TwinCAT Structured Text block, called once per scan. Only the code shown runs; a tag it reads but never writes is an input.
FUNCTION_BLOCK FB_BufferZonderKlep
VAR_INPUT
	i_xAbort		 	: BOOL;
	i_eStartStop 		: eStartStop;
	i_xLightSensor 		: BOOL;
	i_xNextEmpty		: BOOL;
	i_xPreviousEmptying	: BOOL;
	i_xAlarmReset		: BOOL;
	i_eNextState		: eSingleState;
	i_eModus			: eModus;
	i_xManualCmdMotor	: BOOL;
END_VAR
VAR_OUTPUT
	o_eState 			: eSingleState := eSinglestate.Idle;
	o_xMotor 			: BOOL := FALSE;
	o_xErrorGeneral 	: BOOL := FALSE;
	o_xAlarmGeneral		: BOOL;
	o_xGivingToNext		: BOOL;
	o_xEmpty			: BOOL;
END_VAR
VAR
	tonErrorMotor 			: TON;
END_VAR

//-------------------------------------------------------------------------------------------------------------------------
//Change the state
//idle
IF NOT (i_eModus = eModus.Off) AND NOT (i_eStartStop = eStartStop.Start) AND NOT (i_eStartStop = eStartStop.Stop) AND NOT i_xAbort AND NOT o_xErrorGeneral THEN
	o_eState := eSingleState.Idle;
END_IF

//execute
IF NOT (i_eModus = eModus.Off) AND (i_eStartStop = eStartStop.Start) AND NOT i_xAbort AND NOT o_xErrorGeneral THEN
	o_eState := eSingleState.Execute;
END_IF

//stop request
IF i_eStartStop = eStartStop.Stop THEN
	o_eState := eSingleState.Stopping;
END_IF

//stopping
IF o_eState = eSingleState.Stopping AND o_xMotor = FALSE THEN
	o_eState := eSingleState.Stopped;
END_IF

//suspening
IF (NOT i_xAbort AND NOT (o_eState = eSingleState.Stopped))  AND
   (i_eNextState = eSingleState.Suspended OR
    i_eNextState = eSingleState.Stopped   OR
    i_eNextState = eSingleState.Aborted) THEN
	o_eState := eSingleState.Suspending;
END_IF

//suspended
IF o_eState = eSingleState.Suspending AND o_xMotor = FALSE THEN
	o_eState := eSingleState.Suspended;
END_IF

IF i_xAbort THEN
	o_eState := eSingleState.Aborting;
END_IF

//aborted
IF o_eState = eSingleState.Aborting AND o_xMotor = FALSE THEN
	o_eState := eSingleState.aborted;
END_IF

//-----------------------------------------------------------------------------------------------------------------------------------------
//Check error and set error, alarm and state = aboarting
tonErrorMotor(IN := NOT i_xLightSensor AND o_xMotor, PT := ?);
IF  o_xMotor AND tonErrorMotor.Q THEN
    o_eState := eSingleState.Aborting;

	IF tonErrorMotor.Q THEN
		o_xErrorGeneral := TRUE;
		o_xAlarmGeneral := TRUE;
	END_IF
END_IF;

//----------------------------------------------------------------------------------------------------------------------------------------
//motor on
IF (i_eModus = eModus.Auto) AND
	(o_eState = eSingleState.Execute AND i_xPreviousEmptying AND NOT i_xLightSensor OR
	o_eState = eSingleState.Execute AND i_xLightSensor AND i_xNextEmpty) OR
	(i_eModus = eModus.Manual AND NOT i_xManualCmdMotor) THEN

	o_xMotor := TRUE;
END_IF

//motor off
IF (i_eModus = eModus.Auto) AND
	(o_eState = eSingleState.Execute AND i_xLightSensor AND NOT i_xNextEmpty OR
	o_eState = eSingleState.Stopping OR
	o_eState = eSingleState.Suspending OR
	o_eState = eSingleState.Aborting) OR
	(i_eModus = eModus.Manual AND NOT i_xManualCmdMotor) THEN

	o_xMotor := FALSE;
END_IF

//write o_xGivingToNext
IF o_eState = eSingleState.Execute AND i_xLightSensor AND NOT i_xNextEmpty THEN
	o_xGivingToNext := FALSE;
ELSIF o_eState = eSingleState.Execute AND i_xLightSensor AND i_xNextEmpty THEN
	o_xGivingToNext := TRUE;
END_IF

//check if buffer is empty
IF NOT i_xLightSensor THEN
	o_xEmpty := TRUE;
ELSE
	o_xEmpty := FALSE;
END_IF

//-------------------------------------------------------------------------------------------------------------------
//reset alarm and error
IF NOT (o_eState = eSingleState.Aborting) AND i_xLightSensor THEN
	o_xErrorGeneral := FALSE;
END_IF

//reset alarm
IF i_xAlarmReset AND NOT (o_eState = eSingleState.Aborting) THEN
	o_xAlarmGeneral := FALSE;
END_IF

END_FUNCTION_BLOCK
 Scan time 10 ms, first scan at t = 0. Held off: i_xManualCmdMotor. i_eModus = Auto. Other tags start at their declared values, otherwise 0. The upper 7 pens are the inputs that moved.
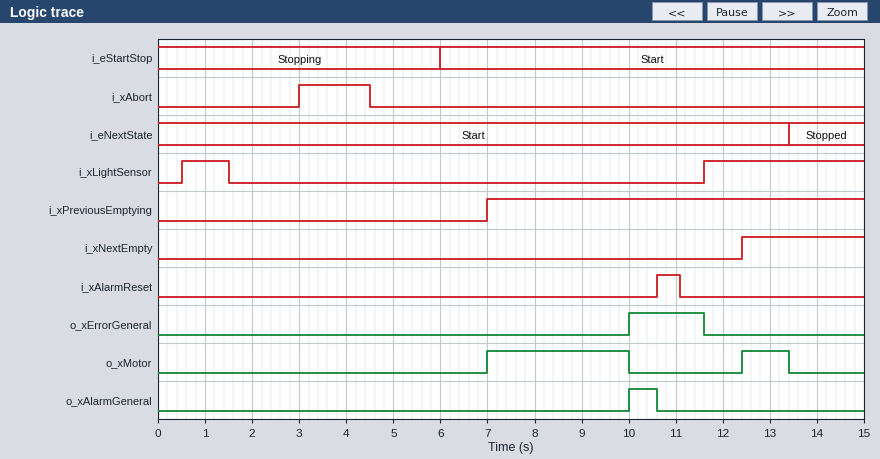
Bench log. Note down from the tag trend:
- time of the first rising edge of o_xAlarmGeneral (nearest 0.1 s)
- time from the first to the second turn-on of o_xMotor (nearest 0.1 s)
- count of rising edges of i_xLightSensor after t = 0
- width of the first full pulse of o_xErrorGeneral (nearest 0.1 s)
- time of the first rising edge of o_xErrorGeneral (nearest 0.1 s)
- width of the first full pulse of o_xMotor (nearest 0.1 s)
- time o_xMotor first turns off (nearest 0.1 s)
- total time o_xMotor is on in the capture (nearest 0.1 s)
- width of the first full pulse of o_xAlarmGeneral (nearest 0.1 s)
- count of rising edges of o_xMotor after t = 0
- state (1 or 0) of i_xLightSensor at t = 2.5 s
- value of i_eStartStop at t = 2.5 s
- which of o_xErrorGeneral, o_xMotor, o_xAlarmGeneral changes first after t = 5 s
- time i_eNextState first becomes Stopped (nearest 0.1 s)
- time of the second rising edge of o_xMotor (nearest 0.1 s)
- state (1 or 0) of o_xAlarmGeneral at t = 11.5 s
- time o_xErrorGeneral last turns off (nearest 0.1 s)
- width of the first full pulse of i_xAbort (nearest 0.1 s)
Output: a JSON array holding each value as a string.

["10.0 s", "5.4 s", "2", "1.6 s", "10.0 s", "3.0 s", "10.0 s", "4.0 s", "0.6 s", "2", "0", "Stopping", "o_xMotor", "13.4 s", "12.4 s", "0", "11.6 s", "1.5 s"]
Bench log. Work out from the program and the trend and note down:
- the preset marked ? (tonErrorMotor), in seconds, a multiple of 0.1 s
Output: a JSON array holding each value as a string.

["3.0 s"]
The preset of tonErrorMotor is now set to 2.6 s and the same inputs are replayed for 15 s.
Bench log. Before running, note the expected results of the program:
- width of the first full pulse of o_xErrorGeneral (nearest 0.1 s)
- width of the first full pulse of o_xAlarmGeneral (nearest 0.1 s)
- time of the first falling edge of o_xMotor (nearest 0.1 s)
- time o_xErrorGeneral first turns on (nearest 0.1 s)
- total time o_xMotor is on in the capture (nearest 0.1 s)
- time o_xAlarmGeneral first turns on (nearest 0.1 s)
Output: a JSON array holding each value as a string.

["2.0 s", "1.0 s", "9.6 s", "9.6 s", "3.6 s", "9.6 s"]
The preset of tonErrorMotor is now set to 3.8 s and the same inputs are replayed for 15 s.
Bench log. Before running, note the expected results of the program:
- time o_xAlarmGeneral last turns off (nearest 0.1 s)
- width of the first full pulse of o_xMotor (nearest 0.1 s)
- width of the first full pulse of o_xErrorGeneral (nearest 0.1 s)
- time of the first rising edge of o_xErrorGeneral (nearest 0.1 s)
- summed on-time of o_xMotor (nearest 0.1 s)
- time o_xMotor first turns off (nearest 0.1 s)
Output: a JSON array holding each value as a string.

["10.8 s", "3.8 s", "0.8 s", "10.8 s", "4.8 s", "10.8 s"]
